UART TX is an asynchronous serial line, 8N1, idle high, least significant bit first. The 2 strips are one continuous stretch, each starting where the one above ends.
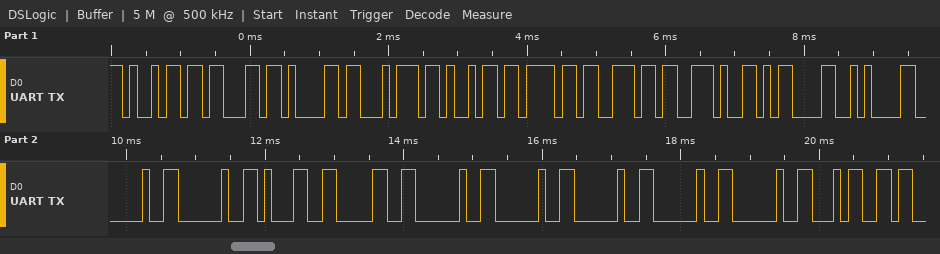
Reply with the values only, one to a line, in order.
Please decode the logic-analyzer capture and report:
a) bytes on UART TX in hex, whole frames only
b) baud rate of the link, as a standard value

69 63 61 74 69 6F 6E 2E 0D 0A 20 20 31 30 20 20 20 20 20 34
9600 baud
